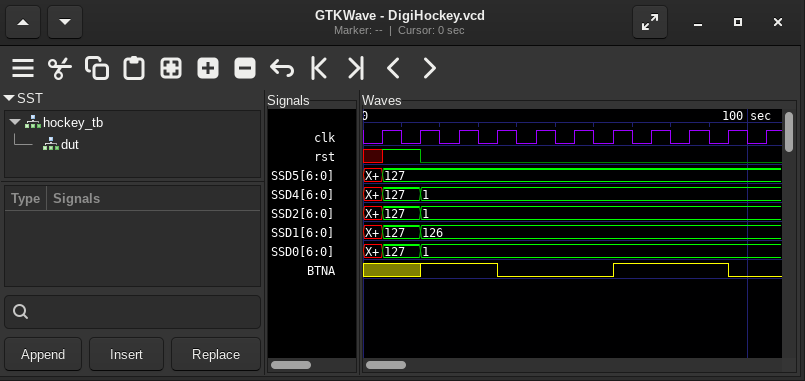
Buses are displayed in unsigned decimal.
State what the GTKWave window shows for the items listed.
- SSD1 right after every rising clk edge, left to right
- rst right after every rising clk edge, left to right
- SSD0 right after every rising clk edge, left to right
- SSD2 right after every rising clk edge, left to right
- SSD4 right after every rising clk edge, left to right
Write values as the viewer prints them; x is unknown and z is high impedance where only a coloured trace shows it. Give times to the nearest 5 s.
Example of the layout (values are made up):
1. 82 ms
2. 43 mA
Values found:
1. 127, 126, 126, 126, 126, 126, 126, 126, 126, 126, 126
2. 1 0 0 0 0 0 0 0 0 0 0
3. 127, 1, 1, 1, 1, 1, 1, 1, 1, 1, 1
4. 127, 1, 1, 1, 1, 1, 1, 1, 1, 1, 1
5. 127, 1, 1, 1, 1, 1, 1, 1, 1, 1, 1
